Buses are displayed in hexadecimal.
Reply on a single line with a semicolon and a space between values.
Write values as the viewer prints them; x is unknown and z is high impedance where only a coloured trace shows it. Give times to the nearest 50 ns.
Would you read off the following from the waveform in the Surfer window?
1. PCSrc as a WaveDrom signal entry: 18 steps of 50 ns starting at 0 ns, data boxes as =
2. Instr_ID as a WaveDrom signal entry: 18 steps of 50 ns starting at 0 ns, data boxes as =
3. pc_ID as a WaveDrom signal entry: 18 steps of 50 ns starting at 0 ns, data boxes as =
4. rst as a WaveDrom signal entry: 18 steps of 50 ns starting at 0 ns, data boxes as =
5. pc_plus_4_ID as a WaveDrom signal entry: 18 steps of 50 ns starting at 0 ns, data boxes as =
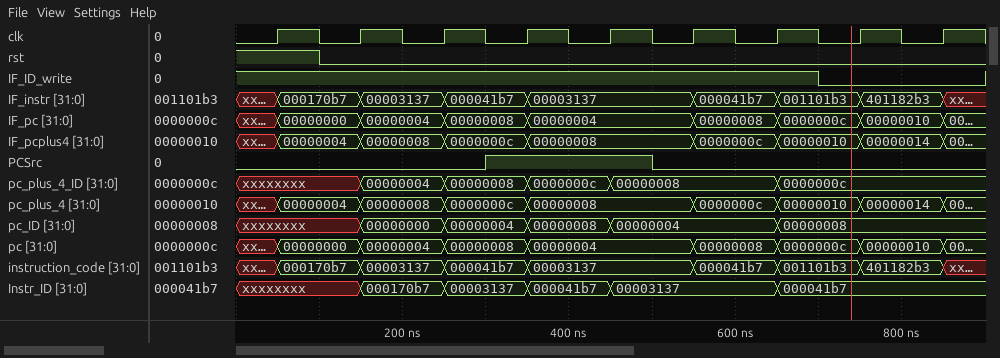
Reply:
{name: 'PCSrc', wave: '0.....1...0.......'}; {name: 'Instr_ID', wave: 'x..=.=.=.=...=....', data: '000170b7 00003137 000041b7 00003137 000041b7'}; {name: 'pc_ID', wave: 'x..=.=.=.=...=....', data: '00000000 00000004 00000008 00000004 00000008'}; {name: 'rst', wave: '1.0...............'}; {name: 'pc_plus_4_ID', wave: 'x..=.=.=.=...=....', data: '00000004 00000008 0000000c 00000008 0000000c'}
